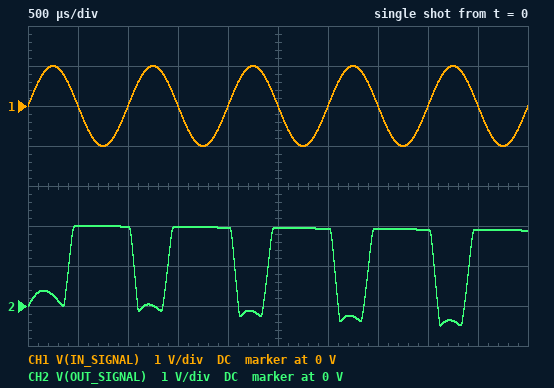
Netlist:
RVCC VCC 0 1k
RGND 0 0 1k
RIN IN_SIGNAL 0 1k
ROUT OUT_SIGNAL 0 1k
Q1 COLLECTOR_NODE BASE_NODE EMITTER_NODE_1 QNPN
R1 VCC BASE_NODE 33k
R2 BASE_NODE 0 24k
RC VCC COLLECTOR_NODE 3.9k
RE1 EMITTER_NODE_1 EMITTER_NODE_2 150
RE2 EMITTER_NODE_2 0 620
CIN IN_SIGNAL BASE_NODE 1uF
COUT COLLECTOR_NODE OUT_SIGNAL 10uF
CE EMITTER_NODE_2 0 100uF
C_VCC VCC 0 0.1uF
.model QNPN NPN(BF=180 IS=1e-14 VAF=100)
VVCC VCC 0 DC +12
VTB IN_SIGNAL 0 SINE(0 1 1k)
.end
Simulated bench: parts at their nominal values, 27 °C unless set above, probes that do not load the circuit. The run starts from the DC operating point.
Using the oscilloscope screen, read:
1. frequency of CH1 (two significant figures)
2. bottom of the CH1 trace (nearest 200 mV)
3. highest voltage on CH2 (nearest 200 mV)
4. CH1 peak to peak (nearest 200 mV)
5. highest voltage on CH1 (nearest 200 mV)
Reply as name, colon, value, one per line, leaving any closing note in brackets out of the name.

frequency of CH1: 1.0 kHz
bottom of the CH1 trace: -1.0 V
highest voltage on CH2: 2.0 V
CH1 peak to peak: 2.0 V
highest voltage on CH1: 1.0 V
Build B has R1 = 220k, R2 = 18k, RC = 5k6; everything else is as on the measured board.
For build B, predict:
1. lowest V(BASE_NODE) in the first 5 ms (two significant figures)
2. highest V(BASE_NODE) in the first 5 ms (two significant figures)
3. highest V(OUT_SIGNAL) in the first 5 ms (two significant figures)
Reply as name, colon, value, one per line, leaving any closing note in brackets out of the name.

lowest V(BASE_NODE) in the first 5 ms: -160 mV
highest V(BASE_NODE) in the first 5 ms: 1.9 V
highest V(OUT_SIGNAL) in the first 5 ms: 380 mV
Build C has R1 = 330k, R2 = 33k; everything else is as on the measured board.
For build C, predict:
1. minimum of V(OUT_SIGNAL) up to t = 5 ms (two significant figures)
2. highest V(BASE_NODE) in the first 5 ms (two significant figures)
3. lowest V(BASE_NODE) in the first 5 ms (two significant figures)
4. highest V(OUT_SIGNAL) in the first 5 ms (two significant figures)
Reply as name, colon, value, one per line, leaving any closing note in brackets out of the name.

minimum of V(OUT_SIGNAL) up to t = 5 ms: -4.8 V
highest V(BASE_NODE) in the first 5 ms: 2.0 V
lowest V(BASE_NODE) in the first 5 ms: -26 mV
highest V(OUT_SIGNAL) in the first 5 ms: 510 mV
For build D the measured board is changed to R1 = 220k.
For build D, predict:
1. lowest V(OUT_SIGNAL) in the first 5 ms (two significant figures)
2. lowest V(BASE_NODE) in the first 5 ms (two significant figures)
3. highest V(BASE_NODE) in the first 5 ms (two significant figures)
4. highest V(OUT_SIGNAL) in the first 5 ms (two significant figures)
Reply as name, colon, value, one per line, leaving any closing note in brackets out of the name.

lowest V(OUT_SIGNAL) in the first 5 ms: -4.8 V
lowest V(BASE_NODE) in the first 5 ms: 71 mV
highest V(BASE_NODE) in the first 5 ms: 2.1 V
highest V(OUT_SIGNAL) in the first 5 ms: 600 mV
